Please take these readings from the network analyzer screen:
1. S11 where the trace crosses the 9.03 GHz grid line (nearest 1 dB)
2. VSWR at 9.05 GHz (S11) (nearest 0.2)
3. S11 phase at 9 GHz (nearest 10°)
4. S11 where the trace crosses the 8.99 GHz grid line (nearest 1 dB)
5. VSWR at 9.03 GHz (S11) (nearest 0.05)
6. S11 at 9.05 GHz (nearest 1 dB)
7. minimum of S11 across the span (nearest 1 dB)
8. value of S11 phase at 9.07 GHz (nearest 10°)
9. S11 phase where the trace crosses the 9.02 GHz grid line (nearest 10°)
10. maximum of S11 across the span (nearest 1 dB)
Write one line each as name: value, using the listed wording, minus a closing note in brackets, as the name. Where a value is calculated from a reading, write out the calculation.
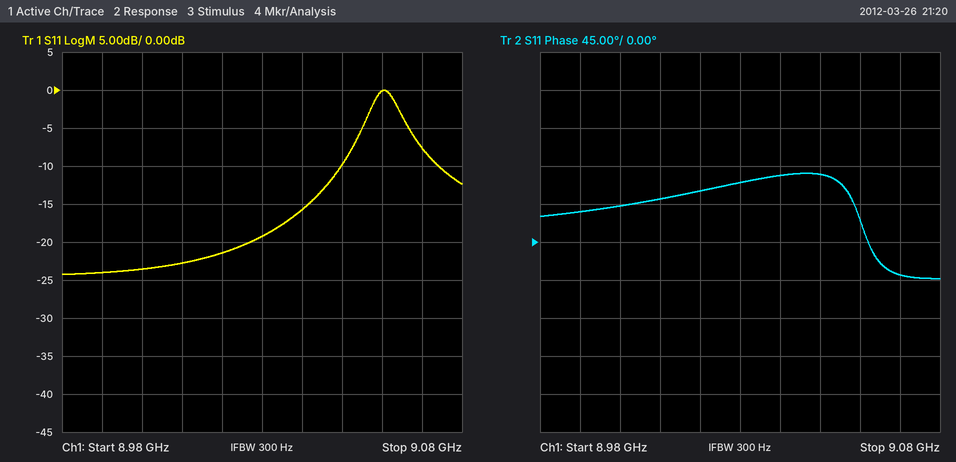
S11 where the trace crosses the 9.03 GHz grid line: -19 dB
VSWR at 9.05 GHz (S11): |Γ| = 10^(-10/20) = 0.3162; VSWR = (1 + 0.3162)/(1 − 0.3162) ≈ 1.92, so 2.0 to the nearest 0.2
S11 phase at 9 GHz: 40°
S11 where the trace crosses the 8.99 GHz grid line: -24 dB
VSWR at 9.03 GHz (S11): |Γ| = 10^(-19/20) = 0.1122; VSWR = (1 + 0.1122)/(1 − 0.1122) ≈ 1.25
S11 at 9.05 GHz: -10 dB
minimum of S11 across the span: -24 dB
value of S11 phase at 9.07 GHz: -40°
S11 phase where the trace crosses the 9.02 GHz grid line: 60°
maximum of S11 across the span: 0 dB
